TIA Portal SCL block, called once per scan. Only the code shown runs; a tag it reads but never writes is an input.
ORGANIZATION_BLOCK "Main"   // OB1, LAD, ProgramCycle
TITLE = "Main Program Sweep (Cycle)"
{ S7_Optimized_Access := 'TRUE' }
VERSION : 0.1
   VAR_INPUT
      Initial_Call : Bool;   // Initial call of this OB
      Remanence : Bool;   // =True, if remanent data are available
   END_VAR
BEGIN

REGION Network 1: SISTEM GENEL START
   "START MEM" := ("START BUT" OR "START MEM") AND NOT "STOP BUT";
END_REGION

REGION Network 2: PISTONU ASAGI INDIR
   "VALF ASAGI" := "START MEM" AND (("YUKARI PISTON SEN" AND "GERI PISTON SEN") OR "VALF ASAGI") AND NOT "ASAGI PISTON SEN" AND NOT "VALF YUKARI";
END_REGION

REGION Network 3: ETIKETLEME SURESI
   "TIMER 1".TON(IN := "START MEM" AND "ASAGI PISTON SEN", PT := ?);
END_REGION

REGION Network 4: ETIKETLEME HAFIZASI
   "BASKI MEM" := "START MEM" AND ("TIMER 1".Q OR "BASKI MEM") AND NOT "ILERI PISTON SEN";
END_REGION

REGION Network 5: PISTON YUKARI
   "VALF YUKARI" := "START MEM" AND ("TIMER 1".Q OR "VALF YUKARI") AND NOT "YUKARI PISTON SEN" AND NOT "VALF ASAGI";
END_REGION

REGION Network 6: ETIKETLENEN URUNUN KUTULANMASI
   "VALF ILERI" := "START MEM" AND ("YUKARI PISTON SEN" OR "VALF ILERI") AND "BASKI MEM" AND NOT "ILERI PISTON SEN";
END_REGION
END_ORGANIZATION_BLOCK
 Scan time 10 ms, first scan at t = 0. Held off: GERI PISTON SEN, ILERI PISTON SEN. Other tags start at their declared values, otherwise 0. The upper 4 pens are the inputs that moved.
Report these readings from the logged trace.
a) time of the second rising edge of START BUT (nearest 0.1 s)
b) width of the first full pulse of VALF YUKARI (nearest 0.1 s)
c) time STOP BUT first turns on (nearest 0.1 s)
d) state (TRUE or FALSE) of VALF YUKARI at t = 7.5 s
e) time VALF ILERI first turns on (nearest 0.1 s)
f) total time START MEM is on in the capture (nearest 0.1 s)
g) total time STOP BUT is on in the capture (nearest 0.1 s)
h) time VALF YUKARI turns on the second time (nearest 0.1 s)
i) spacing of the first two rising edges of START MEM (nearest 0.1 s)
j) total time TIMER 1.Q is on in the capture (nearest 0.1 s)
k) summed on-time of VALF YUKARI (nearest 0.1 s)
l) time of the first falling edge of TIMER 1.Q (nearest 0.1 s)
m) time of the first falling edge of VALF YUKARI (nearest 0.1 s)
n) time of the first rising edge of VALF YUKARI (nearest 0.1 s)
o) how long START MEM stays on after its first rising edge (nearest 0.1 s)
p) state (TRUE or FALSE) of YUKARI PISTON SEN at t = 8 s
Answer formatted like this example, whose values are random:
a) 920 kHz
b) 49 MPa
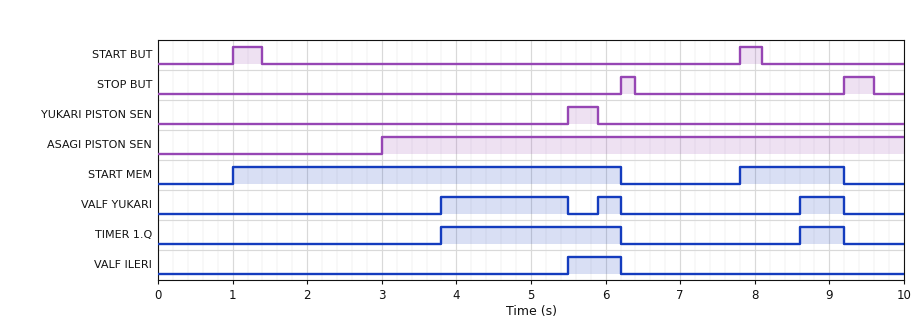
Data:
a) 7.8 s
b) 1.7 s
c) 6.2 s
d) FALSE
e) 5.5 s
f) 6.6 s
g) 0.6 s
h) 5.9 s
i) 6.8 s
j) 3.0 s
k) 2.6 s
l) 6.2 s
m) 5.5 s
n) 3.8 s
o) 5.2 s
p) FALSE
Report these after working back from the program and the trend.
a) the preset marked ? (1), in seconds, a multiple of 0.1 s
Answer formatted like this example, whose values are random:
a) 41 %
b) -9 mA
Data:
a) 0.8 s
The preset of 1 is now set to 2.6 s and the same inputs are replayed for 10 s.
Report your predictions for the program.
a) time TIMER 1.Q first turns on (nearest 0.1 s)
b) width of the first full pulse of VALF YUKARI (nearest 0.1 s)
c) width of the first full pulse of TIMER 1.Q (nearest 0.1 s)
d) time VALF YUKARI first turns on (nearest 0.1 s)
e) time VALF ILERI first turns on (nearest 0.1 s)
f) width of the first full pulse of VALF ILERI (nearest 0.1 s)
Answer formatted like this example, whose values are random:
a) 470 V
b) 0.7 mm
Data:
a) 5.6 s
b) 0.3 s
c) 0.6 s
d) 5.9 s
e) 5.6 s
f) 0.6 s
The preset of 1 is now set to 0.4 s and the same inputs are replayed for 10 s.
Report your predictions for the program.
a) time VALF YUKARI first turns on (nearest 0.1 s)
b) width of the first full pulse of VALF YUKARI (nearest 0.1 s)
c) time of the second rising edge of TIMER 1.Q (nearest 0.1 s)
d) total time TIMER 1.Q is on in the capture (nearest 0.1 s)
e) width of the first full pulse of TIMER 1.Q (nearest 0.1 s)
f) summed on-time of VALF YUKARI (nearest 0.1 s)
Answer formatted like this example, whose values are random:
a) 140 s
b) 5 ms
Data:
a) 3.4 s
b) 2.1 s
c) 8.2 s
d) 3.8 s
e) 2.8 s
f) 3.4 s
